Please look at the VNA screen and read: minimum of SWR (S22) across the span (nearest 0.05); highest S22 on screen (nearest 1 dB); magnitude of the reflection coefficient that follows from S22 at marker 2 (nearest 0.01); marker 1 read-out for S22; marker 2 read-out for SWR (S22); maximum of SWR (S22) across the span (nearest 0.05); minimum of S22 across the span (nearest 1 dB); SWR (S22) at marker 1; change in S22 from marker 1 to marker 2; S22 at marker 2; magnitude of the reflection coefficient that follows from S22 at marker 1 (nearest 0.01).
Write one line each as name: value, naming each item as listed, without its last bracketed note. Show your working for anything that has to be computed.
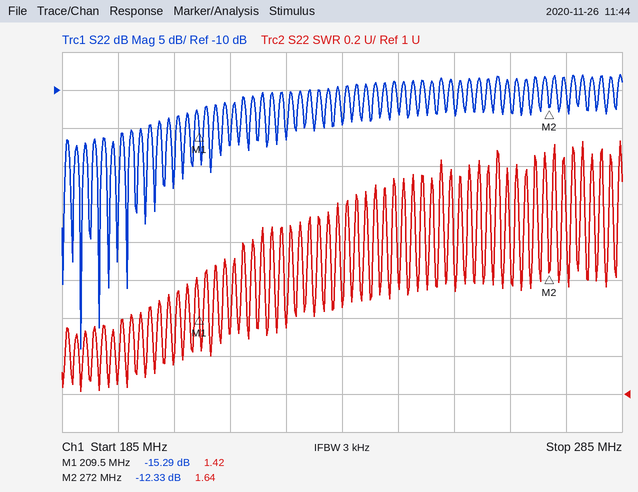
minimum of SWR (S22) across the span: 1.00
highest S22 on screen: -8 dB
magnitude of the reflection coefficient that follows from S22 at marker 2: 10^(-12.33/20) ≈ 0.24
marker 1 read-out for S22: -15.29 dB
marker 2 read-out for SWR: 1.64
maximum of SWR (S22) across the span: 2.35
minimum of S22 across the span: -44 dB
SWR (S22) at marker 1: 1.42
change in S22 from marker 1 to marker 2: -12.33 − (-15.29) = 2.96 dB
S22 at marker 2: -12.33 dB
magnitude of the reflection coefficient that follows from S22 at marker 1: 10^(-15.29/20) ≈ 0.17
